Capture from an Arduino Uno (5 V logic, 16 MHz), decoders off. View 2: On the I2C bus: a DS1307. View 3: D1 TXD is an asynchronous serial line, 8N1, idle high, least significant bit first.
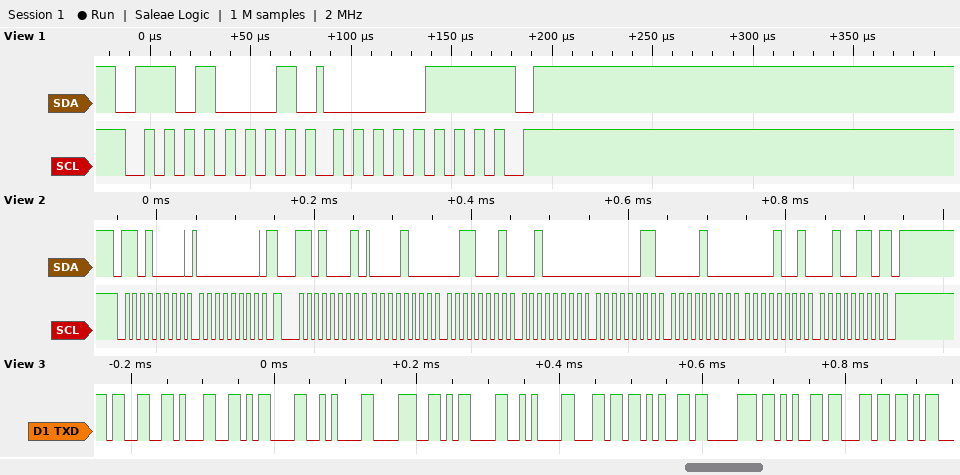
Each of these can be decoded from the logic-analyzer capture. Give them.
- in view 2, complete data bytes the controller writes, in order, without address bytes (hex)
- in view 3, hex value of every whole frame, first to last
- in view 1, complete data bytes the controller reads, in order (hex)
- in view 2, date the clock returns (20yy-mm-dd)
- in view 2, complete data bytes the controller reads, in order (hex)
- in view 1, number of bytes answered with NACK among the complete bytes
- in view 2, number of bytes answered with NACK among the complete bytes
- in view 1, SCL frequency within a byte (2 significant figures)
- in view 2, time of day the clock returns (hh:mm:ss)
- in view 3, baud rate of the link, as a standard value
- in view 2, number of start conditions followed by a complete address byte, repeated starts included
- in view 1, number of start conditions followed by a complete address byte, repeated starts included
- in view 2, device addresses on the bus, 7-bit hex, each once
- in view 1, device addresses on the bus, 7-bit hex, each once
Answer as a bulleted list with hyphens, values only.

- 00
- 33 31 0D 0A 38 0D 0A 6C 65 70 65 6C
- 07
- 2026-09-08
- 08 31 20 03 08 09 26
- 1
- 1
- 100 kHz
- 20:31:08
- 115200 baud
- 2
- 1
- 0x68
- 0x68
